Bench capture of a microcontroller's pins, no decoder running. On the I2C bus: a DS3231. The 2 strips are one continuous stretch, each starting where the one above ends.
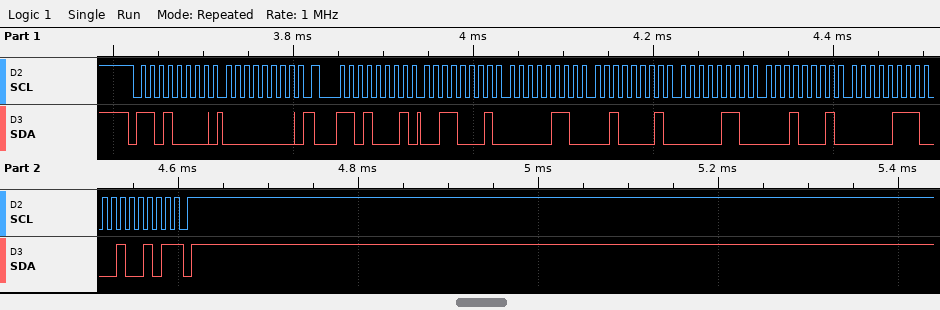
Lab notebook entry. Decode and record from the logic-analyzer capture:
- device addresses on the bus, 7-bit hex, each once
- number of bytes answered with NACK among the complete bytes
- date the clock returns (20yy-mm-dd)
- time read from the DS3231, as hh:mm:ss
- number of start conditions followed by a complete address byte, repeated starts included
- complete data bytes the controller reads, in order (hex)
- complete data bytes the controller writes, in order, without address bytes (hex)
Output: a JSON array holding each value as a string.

["0x68", "1", "2025-07-11", "21:06:31", "2", "31 06 21 06 11 07 25", "00"]
